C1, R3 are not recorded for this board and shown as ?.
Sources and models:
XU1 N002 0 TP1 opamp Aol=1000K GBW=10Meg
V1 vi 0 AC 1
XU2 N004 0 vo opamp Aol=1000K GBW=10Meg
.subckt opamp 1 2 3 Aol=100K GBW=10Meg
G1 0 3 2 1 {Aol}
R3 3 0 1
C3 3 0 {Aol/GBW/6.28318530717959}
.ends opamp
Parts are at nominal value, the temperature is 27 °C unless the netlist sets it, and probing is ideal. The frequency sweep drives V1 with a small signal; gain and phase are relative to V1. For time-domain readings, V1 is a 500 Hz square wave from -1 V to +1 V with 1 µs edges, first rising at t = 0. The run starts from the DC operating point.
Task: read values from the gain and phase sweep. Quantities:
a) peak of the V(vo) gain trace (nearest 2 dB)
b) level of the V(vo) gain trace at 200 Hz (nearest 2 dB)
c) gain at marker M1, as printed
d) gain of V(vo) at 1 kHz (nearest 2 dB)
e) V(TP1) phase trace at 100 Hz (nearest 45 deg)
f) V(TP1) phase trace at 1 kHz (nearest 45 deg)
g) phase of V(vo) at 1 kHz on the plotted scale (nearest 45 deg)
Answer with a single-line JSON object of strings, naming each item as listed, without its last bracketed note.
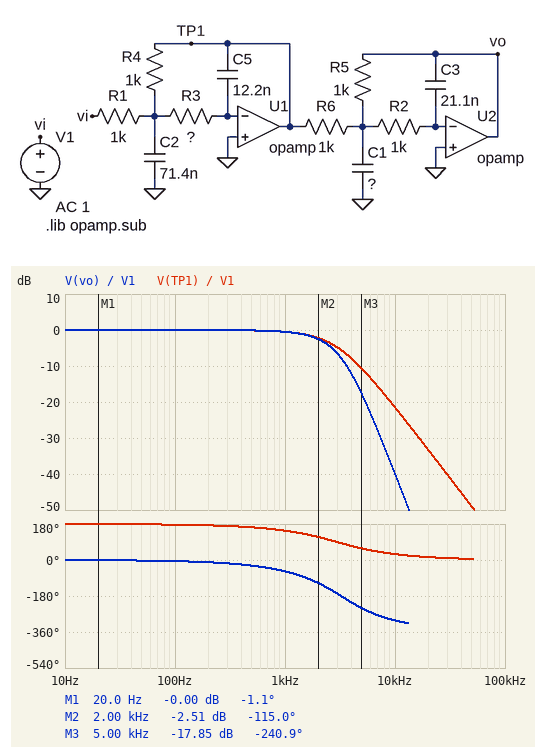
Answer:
{"peak of the V(vo) gain trace": "0 dB", "level of the V(vo) gain trace at 200 Hz": "0 dB", "gain at marker M1, as printed": "-0.00 dB", "gain of V(vo) at 1 kHz": "0 dB", "V(TP1) phase trace at 100 Hz": "180 deg", "V(TP1) phase trace at 1 kHz": "135 deg", "phase of V(vo) at 1 kHz on the plotted scale": "-45 deg"}
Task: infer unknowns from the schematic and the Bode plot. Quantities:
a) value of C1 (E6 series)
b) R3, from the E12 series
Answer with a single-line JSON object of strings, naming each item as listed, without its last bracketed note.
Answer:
{"value of C1": "100 nF", "R3, from the E12 series": "3.3 kΩ"}
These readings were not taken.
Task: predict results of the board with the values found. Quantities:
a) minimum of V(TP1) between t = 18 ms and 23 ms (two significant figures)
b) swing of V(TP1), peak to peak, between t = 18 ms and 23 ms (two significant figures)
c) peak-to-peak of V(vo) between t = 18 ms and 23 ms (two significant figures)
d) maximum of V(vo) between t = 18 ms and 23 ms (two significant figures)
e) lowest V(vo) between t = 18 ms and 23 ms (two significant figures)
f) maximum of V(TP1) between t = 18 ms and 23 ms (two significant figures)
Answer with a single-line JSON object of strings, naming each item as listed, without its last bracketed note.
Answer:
{"minimum of V(TP1) between t = 18 ms and 23 ms": "-1.0 V", "swing of V(TP1), peak to peak, between t = 18 ms and 23 ms": "2.0 V", "peak-to-peak of V(vo) between t = 18 ms and 23 ms": "2.1 V", "maximum of V(vo) between t = 18 ms and 23 ms": "1.0 V", "lowest V(vo) between t = 18 ms and 23 ms": "-1.0 V", "maximum of V(TP1) between t = 18 ms and 23 ms": "1.0 V"}
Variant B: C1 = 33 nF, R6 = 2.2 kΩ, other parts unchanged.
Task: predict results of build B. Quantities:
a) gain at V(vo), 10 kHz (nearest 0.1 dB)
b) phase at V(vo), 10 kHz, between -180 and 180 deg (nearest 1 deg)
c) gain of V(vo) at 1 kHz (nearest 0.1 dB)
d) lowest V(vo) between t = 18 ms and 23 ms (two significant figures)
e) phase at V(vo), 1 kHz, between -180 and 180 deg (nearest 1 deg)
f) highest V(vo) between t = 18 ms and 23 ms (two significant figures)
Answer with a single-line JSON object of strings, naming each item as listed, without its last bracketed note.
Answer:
{"gain at V(vo), 10 kHz": "-39.7 dB", "phase at V(vo), 10 kHz, between -180 and 180 deg": "91 deg", "gain of V(vo) at 1 kHz": "-7.6 dB", "lowest V(vo) between t = 18 ms and 23 ms": "-460 mV", "phase at V(vo), 1 kHz, between -180 and 180 deg": "-52 deg", "highest V(vo) between t = 18 ms and 23 ms": "460 mV"}
